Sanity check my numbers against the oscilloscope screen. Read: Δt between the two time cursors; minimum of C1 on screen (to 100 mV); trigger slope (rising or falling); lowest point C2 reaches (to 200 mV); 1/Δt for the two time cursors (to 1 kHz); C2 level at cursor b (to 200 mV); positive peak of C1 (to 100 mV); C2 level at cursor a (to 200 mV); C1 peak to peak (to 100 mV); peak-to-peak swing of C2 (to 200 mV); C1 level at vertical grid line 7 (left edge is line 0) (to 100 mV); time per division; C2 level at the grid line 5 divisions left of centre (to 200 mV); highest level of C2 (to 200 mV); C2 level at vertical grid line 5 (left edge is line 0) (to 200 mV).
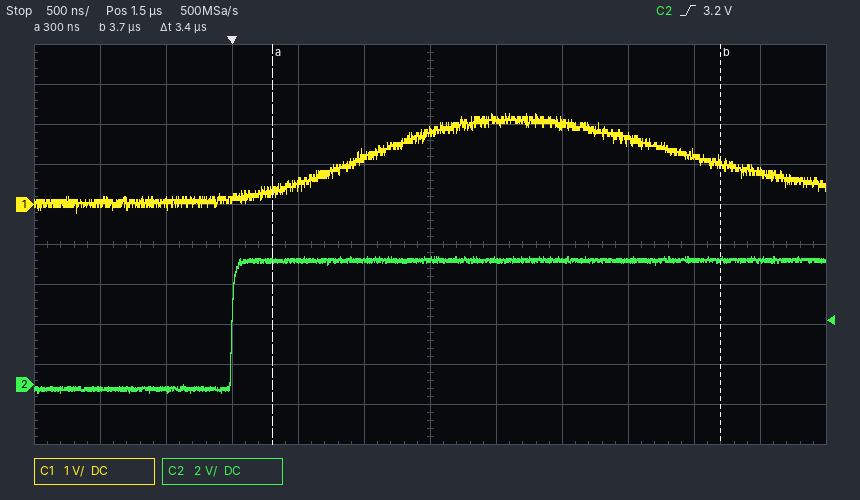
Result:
3.4 µs
-200 mV
rising
-400 mV
294 kHz
6.2 V
2.3 V
6.2 V
2.5 V
6.8 V
2.1 V
500 ns
-200 mV
6.4 V
6.2 V
